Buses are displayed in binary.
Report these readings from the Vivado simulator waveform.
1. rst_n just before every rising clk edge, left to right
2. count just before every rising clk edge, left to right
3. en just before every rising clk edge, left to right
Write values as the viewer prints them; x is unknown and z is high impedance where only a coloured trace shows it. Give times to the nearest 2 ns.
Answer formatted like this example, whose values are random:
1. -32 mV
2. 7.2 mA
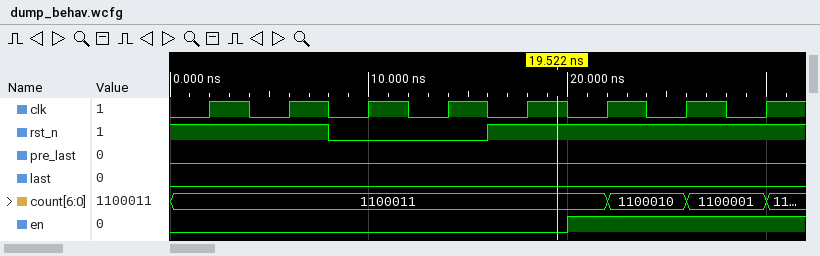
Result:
1. 1 1 0 0 1 1 1 1
2. 1100011, 1100011, 1100011, 1100011, 1100011, 1100011, 1100010, 1100001
3. 0 0 0 0 0 1 1 1
